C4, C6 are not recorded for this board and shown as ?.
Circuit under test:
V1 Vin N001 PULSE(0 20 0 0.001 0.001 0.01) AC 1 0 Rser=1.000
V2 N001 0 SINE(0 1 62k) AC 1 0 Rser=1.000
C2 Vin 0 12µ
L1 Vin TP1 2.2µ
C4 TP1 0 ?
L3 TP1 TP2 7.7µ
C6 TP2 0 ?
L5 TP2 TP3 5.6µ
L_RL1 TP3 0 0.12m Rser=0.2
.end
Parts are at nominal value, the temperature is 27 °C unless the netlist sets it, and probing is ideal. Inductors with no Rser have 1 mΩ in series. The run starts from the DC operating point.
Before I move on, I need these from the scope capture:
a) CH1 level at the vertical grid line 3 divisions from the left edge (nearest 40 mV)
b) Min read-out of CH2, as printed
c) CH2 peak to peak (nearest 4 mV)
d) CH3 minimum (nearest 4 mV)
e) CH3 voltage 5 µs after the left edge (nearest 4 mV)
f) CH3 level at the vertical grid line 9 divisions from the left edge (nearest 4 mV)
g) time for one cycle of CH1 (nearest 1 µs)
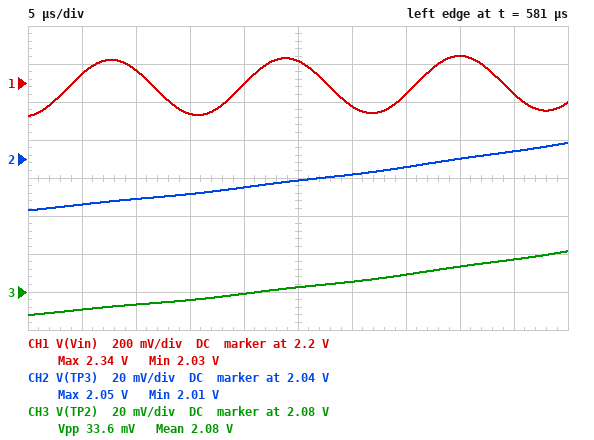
2.04 V
2.01 V
36 mV
2.068 V
2.072 V
2.096 V
16 µs
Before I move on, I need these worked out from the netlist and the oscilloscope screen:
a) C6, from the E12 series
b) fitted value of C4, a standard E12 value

56 µF
27 µF
